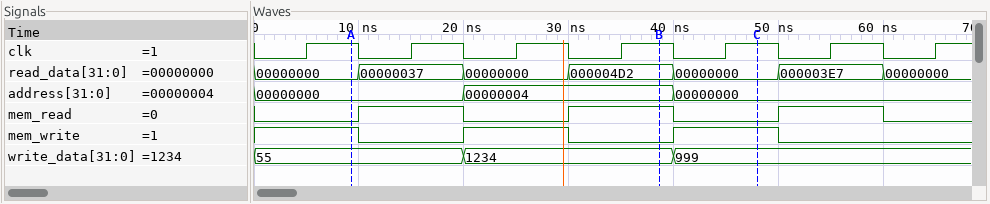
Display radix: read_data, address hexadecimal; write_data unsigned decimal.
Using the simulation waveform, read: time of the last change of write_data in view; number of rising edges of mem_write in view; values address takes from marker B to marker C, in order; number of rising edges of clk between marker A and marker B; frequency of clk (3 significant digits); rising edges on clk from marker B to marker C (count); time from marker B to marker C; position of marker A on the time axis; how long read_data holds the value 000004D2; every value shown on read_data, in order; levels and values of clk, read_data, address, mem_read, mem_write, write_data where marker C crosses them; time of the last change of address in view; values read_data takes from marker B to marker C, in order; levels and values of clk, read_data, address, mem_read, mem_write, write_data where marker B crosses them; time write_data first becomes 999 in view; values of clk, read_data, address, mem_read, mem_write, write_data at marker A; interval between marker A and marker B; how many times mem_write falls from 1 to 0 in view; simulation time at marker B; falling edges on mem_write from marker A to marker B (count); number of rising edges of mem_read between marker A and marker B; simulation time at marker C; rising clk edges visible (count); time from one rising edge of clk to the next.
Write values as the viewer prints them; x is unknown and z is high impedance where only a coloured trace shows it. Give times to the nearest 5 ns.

40 ns
2
00000004, 00000000
3
100 MHz
1
10 ns
10 ns
10 ns
00000000, 00000037, 00000000, 000004D2, 00000000, 000003E7, 00000000
clk=1, read_data=00000000, address=00000000, mem_read=0, mem_write=1, write_data=999
40 ns
000004D2, 00000000
clk=1, read_data=000004D2, address=00000004, mem_read=1, mem_write=0, write_data=1234
40 ns
clk=1, read_data=00000000, address=00000000, mem_read=0, mem_write=1, write_data=55
30 ns
3
40 ns
2
2
50 ns
7
10 ns
